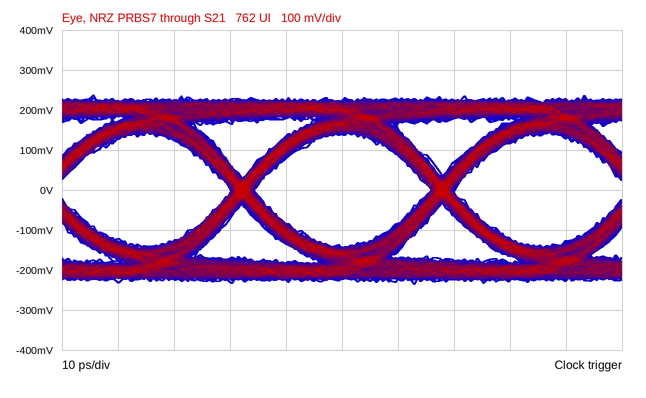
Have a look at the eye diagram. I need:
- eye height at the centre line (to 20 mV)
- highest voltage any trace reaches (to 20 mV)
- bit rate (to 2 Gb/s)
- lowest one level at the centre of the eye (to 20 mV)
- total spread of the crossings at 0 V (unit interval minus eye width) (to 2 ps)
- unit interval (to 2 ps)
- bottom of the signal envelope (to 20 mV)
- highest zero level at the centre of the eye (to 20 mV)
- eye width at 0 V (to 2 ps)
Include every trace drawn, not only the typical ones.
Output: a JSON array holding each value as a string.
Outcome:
["280 mV", "240 mV", "28 Gb/s", "140 mV", "4 ps", "36 ps", "-240 mV", "-140 mV", "32 ps"]
